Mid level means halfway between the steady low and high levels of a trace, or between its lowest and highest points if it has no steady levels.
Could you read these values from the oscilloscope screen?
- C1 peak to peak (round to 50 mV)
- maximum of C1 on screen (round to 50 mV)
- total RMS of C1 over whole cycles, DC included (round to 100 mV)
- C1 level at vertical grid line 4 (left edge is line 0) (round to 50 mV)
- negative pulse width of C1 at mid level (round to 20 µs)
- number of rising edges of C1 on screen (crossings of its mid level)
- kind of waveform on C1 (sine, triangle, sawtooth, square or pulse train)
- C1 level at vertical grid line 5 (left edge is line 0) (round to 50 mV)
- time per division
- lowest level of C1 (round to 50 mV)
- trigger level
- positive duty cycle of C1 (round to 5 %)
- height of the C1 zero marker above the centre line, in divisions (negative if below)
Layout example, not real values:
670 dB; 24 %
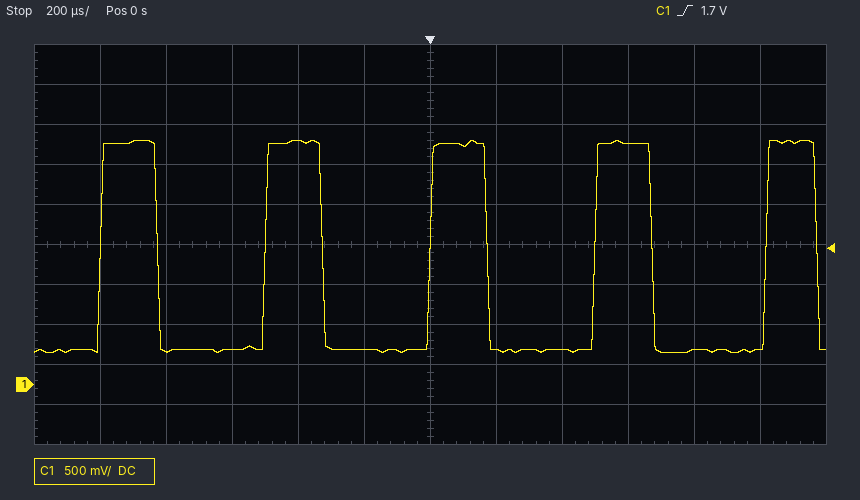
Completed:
2.65 V; 3.05 V; 1.8 V; 3.05 V; 340 µs; 5; pulse train; 450 mV; 200 µs; 400 mV; 1.7 V; 35 %; -3.5 div
